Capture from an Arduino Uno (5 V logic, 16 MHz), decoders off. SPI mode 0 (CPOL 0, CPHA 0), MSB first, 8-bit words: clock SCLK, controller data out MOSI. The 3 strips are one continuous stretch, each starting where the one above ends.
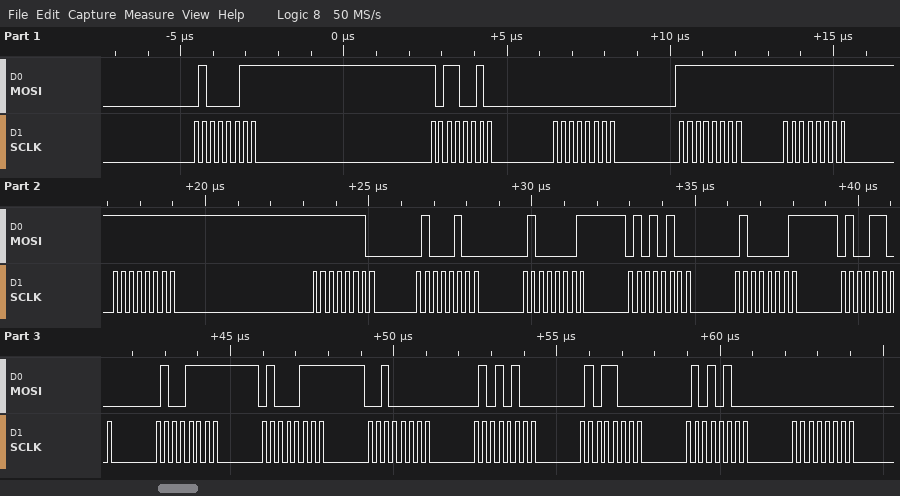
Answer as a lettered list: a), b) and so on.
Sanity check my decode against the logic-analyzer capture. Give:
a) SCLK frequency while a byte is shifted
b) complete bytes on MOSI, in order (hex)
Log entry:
a) 4 MHz
b) 43 B2 00 FF FF FF FE 44 41 54 41 4C 4F 47 20 54 58 54 00
